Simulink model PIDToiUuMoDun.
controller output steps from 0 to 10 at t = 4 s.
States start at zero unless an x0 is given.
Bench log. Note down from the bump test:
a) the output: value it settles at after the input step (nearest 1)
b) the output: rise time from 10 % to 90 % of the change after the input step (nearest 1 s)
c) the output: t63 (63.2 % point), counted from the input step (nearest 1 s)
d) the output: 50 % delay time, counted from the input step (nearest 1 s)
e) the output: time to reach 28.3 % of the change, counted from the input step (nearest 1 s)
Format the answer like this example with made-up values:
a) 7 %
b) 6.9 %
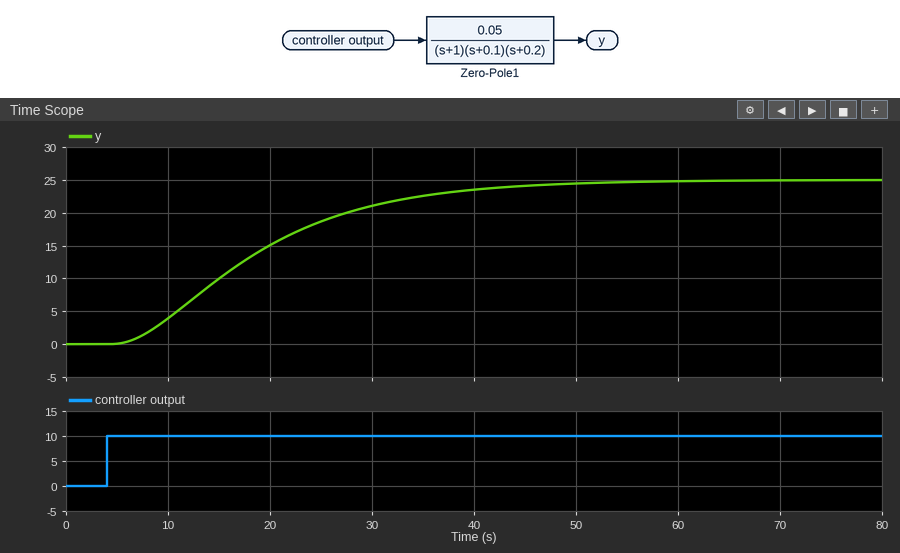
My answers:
a) 25
b) 26 s
c) 17 s
d) 13 s
e) 9 s
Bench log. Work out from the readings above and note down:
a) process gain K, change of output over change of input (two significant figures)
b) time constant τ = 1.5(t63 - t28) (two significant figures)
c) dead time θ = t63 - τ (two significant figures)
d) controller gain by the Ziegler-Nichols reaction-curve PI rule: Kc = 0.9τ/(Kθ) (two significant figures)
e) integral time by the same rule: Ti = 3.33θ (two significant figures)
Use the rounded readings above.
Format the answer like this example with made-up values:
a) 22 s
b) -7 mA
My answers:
a) 2.5
b) 12 s
c) 5.0 s
d) 0.86
e) 17 s
